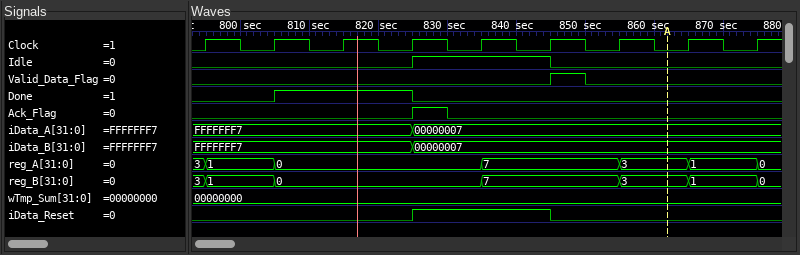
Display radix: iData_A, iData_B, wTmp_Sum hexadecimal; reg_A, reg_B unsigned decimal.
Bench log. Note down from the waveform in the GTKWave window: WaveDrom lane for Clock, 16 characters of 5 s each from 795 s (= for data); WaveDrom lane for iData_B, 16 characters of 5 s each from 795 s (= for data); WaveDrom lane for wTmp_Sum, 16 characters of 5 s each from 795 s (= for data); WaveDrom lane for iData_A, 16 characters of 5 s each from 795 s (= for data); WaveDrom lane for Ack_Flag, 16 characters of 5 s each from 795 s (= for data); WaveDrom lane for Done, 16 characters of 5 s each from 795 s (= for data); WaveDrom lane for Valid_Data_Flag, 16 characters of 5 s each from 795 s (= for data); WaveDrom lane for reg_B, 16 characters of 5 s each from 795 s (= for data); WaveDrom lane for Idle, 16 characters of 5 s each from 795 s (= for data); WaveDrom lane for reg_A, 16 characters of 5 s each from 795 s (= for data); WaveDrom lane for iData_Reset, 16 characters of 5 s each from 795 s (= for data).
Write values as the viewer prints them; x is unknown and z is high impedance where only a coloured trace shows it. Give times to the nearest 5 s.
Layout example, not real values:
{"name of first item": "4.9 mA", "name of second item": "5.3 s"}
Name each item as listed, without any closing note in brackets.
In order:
{"WaveDrom lane for Clock, 16 characters of 5 s each from 795 s": "{name: 'Clock', wave: '1010101010101010'}", "WaveDrom lane for iData_B, 16 characters of 5 s each from 795 s": "{name: 'iData_B', wave: '=.....=.........', data: 'FFFFFFF7 00000007'}", "WaveDrom lane for wTmp_Sum, 16 characters of 5 s each from 795 s": "{name: 'wTmp_Sum', wave: '=...............', data: '00000000'}", "WaveDrom lane for iData_A, 16 characters of 5 s each from 795 s": "{name: 'iData_A', wave: '=.....=.........', data: 'FFFFFFF7 00000007'}", "WaveDrom lane for Ack_Flag, 16 characters of 5 s each from 795 s": "{name: 'Ack_Flag', wave: '0.....10........'}", "WaveDrom lane for Done, 16 characters of 5 s each from 795 s": "{name: 'Done', wave: '0.1...0.........'}", "WaveDrom lane for Valid_Data_Flag, 16 characters of 5 s each from 795 s": "{name: 'Valid_Data_Flag', wave: '0.........10....'}", "WaveDrom lane for reg_B, 16 characters of 5 s each from 795 s": "{name: 'reg_B', wave: '=.=.....=...=.=.', data: '1 0 7 3 1'}", "WaveDrom lane for Idle, 16 characters of 5 s each from 795 s": "{name: 'Idle', wave: '0.....1...0.....'}", "WaveDrom lane for reg_A, 16 characters of 5 s each from 795 s": "{name: 'reg_A', wave: '=.=.....=...=.=.', data: '1 0 7 3 1'}", "WaveDrom lane for iData_Reset, 16 characters of 5 s each from 795 s": "{name: 'iData_Reset', wave: '0.....1...0.....'}"}
